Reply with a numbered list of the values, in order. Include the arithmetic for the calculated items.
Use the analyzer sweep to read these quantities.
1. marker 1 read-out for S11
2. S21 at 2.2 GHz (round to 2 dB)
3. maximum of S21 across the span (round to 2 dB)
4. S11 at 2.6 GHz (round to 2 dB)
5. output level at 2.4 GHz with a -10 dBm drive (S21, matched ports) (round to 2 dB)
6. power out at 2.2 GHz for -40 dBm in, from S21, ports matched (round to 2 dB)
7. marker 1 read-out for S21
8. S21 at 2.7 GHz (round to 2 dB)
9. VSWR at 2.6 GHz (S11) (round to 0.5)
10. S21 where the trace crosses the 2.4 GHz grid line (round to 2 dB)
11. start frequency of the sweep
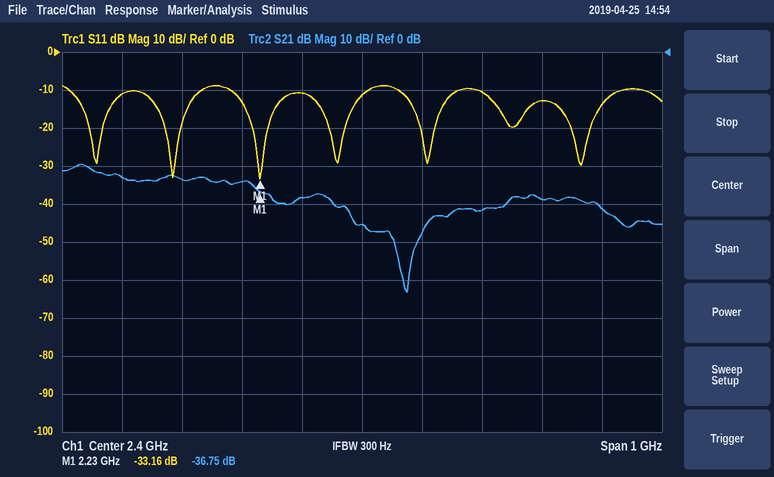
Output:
1. -33.16 dB
2. -34 dB
3. -30 dB
4. -10 dB
5. -10 dBm + (-46 dB) = -56 dBm
6. -40 dBm + (-34 dB) = -74 dBm
7. -36.75 dB
8. -38 dB
9. |Γ| = 10^(-10/20) = 0.3162; VSWR = (1 + 0.3162)/(1 − 0.3162) ≈ 1.92, so 2.0 to the nearest 0.5
10. -46 dB
11. 1.9 GHz
